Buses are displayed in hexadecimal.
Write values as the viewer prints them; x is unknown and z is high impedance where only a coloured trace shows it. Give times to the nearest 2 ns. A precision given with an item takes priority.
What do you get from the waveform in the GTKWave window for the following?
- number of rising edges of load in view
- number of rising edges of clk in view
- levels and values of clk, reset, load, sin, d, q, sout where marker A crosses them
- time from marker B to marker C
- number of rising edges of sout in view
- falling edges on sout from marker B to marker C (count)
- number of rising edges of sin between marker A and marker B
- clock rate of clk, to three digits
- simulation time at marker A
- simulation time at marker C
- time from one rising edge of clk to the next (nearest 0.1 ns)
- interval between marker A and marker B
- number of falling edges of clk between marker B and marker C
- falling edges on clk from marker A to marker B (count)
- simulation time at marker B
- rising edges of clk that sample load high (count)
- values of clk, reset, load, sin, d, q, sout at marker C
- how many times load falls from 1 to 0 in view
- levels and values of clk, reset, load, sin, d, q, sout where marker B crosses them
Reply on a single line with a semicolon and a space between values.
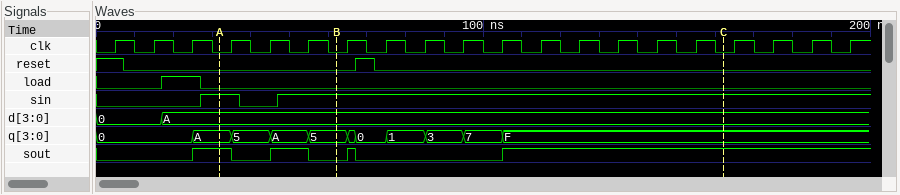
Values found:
1; 20; clk=0, reset=0, load=0, sin=1, d=A, q=A, sout=1; 100 ns; 4; 1; 1; 100 MHz; 32 ns; 162 ns; 10 ns; 30 ns; 10; 3; 62 ns; 1; clk=0, reset=0, load=0, sin=1, d=A, q=F, sout=1; 1; clk=0, reset=0, load=0, sin=1, d=A, q=5, sout=0
